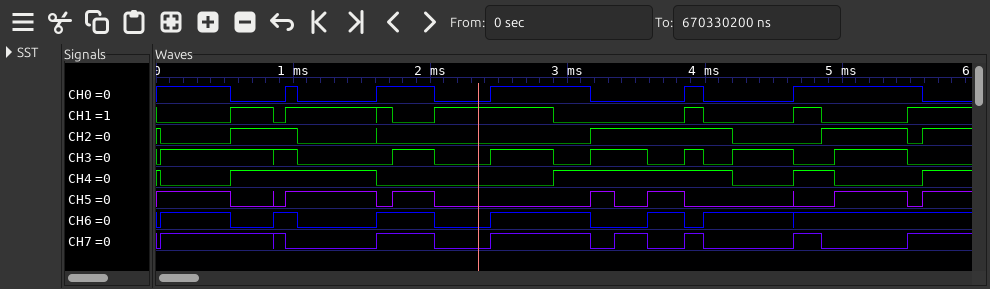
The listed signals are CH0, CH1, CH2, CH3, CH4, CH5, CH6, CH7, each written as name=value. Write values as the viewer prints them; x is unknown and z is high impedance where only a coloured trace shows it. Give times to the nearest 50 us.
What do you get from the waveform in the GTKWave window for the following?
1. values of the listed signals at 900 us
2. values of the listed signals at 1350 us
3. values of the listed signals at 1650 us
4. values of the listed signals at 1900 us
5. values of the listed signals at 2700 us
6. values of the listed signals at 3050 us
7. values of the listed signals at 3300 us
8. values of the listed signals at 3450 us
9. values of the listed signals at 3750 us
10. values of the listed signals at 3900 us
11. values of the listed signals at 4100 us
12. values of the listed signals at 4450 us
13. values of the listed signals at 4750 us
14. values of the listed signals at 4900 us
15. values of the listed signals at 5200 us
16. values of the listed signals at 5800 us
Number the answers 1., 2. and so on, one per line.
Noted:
1. CH0=0, CH1=0, CH2=1, CH3=1, CH4=1, CH5=0, CH6=1, CH7=1
2. CH0=0, CH1=1, CH2=0, CH3=0, CH4=1, CH5=1, CH6=0, CH7=0
3. CH0=1, CH1=1, CH2=0, CH3=0, CH4=0, CH5=0, CH6=1, CH7=1
4. CH0=1, CH1=0, CH2=0, CH3=1, CH4=0, CH5=1, CH6=1, CH7=1
5. CH0=1, CH1=1, CH2=0, CH3=1, CH4=0, CH5=0, CH6=1, CH7=1
6. CH0=1, CH1=0, CH2=0, CH3=0, CH4=1, CH5=0, CH6=1, CH7=1
7. CH0=0, CH1=0, CH2=1, CH3=1, CH4=1, CH5=1, CH6=0, CH7=0
8. CH0=0, CH1=0, CH2=1, CH3=1, CH4=1, CH5=0, CH6=0, CH7=1
9. CH0=0, CH1=0, CH2=1, CH3=0, CH4=1, CH5=1, CH6=1, CH7=0
10. CH0=1, CH1=1, CH2=1, CH3=1, CH4=1, CH5=0, CH6=0, CH7=1
11. CH0=0, CH1=0, CH2=1, CH3=0, CH4=1, CH5=0, CH6=1, CH7=0
12. CH0=0, CH1=0, CH2=0, CH3=1, CH4=0, CH5=0, CH6=1, CH7=0
13. CH0=1, CH1=1, CH2=0, CH3=0, CH4=1, CH5=0, CH6=1, CH7=1
14. CH0=1, CH1=0, CH2=1, CH3=0, CH4=1, CH5=0, CH6=1, CH7=0
15. CH0=1, CH1=0, CH2=1, CH3=1, CH4=0, CH5=1, CH6=1, CH7=0
16. CH0=0, CH1=1, CH2=1, CH3=0, CH4=1, CH5=1, CH6=1, CH7=1
